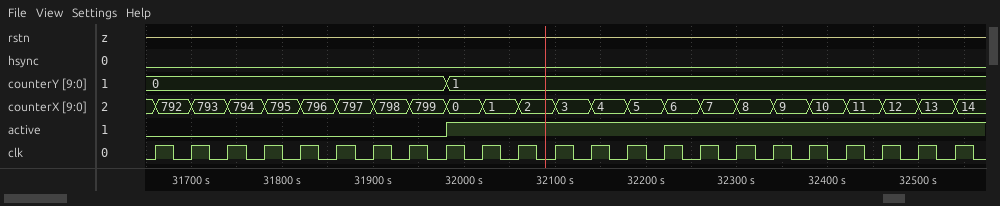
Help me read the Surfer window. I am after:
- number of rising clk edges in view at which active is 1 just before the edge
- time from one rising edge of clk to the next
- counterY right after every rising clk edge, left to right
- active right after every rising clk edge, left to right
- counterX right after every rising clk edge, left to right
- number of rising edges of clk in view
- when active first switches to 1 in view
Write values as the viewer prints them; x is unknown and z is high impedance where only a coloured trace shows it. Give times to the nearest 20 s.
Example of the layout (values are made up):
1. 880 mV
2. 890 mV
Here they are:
1. 14
2. 40 s
3. 0, 0, 0, 0, 0, 0, 0, 0, 1, 1, 1, 1, 1, 1, 1, 1, 1, 1, 1, 1, 1, 1, 1
4. 0 0 0 0 0 0 0 0 1 1 1 1 1 1 1 1 1 1 1 1 1 1 1
5. 792, 793, 794, 795, 796, 797, 798, 799, 0, 1, 2, 3, 4, 5, 6, 7, 8, 9, 10, 11, 12, 13, 14
6. 23
7. 31980 s
